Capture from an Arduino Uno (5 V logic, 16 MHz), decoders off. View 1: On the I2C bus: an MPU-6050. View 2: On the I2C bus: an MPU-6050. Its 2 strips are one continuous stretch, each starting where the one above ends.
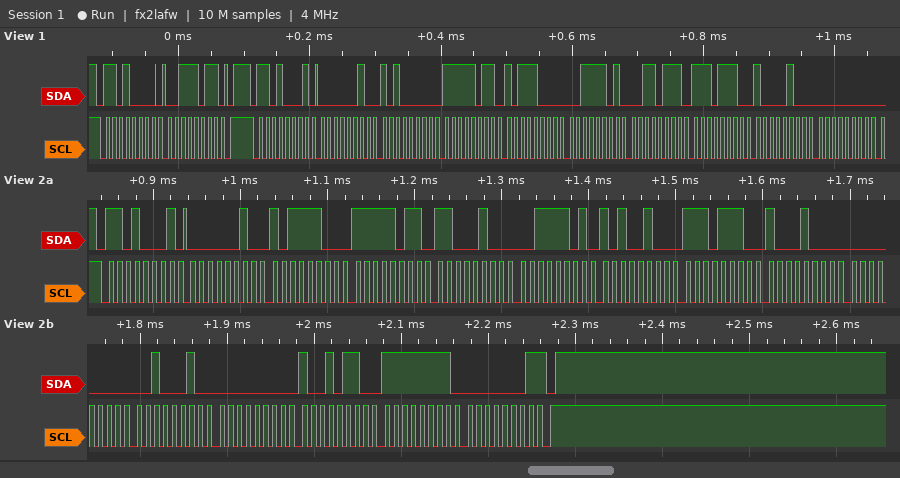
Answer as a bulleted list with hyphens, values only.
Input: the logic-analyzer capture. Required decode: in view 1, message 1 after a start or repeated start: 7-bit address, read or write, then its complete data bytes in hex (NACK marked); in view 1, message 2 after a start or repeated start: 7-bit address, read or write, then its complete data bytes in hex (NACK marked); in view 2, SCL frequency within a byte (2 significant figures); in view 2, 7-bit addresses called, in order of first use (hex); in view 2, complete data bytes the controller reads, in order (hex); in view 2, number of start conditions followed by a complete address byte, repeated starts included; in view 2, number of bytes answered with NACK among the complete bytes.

- 0x68 write: 3B
- 0x68 read: 02 A0 FB B8 3D 37 EE 84 00
- 100 kHz
- 0x68
- 02 BC FB C4 3D A4 EE 88 00 22 00 96 FF 01
- 1
- 1
